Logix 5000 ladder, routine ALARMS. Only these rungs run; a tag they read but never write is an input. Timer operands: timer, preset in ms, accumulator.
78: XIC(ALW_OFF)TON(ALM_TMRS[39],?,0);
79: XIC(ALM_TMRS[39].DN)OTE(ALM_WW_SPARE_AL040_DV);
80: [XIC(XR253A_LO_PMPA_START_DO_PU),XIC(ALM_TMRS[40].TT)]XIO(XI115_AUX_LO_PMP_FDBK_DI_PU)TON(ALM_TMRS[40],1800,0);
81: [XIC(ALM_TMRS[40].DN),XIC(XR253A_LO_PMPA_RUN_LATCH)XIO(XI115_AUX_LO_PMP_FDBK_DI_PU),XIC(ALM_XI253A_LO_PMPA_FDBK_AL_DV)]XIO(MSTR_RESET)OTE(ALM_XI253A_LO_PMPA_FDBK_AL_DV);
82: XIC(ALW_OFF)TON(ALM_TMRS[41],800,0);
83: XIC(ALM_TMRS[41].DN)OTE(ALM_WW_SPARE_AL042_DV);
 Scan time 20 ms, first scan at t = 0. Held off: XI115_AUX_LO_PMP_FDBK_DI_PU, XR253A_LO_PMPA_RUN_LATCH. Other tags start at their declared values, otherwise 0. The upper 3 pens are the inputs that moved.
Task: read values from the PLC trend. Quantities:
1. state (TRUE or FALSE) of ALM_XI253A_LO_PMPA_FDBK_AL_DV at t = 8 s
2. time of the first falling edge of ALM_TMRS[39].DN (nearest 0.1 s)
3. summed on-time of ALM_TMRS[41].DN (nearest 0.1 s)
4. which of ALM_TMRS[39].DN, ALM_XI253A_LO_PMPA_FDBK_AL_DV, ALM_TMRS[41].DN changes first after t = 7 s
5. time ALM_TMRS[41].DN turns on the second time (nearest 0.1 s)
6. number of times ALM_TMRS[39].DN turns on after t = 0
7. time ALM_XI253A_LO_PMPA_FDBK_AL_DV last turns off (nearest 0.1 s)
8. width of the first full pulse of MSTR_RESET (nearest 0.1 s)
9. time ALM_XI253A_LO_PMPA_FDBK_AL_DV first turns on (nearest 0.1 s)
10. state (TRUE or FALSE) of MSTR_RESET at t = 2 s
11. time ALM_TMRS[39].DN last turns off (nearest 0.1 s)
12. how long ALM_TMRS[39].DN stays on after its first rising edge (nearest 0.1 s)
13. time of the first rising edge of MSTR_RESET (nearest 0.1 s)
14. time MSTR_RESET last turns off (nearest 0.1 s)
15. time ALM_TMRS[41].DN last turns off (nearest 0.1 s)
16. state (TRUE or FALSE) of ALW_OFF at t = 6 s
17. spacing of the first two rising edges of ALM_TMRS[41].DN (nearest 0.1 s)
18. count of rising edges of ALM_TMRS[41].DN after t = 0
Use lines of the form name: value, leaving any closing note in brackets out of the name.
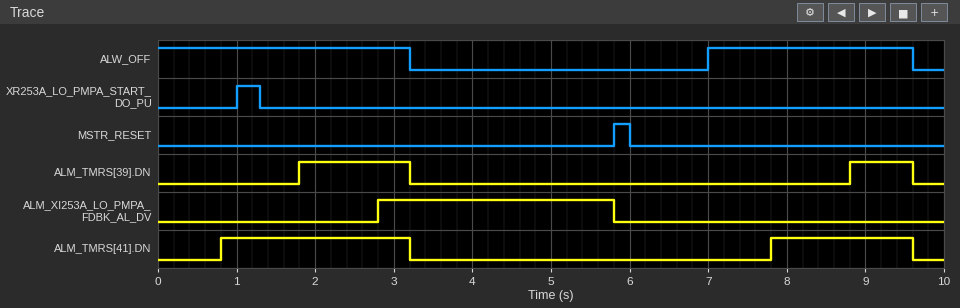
state (TRUE or FALSE) of ALM_XI253A_LO_PMPA_FDBK_AL_DV at t = 8 s: FALSE
time of the first falling edge of ALM_TMRS[39].DN: 3.2 s
summed on-time of ALM_TMRS[41].DN: 4.2 s
which of ALM_TMRS[39].DN, ALM_XI253A_LO_PMPA_FDBK_AL_DV, ALM_TMRS[41].DN changes first after t = 7 s: ALM_TMRS[41].DN
time ALM_TMRS[41].DN turns on the second time: 7.8 s
number of times ALM_TMRS[39].DN turns on after t = 0: 2
time ALM_XI253A_LO_PMPA_FDBK_AL_DV last turns off: 5.8 s
width of the first full pulse of MSTR_RESET: 0.2 s
time ALM_XI253A_LO_PMPA_FDBK_AL_DV first turns on: 2.8 s
state (TRUE or FALSE) of MSTR_RESET at t = 2 s: FALSE
time ALM_TMRS[39].DN last turns off: 9.6 s
how long ALM_TMRS[39].DN stays on after its first rising edge: 1.4 s
time of the first rising edge of MSTR_RESET: 5.8 s
time MSTR_RESET last turns off: 6.0 s
time ALM_TMRS[41].DN last turns off: 9.6 s
state (TRUE or FALSE) of ALW_OFF at t = 6 s: FALSE
spacing of the first two rising edges of ALM_TMRS[41].DN: 7.0 s
count of rising edges of ALM_TMRS[41].DN after t = 0: 2
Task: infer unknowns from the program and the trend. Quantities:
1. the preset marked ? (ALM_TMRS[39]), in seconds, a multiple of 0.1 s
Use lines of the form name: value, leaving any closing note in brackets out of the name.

the preset marked ? (ALM_TMRS[39]), in seconds, a multiple of 0.1 s: 1.8 s
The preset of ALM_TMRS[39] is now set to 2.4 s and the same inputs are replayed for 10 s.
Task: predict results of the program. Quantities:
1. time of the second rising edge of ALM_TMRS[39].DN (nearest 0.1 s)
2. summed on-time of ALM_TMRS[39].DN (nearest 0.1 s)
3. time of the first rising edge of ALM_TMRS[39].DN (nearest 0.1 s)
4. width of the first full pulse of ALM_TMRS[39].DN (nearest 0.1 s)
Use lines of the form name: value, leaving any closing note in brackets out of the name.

time of the second rising edge of ALM_TMRS[39].DN: 9.4 s
summed on-time of ALM_TMRS[39].DN: 1.0 s
time of the first rising edge of ALM_TMRS[39].DN: 2.4 s
width of the first full pulse of ALM_TMRS[39].DN: 0.8 s
